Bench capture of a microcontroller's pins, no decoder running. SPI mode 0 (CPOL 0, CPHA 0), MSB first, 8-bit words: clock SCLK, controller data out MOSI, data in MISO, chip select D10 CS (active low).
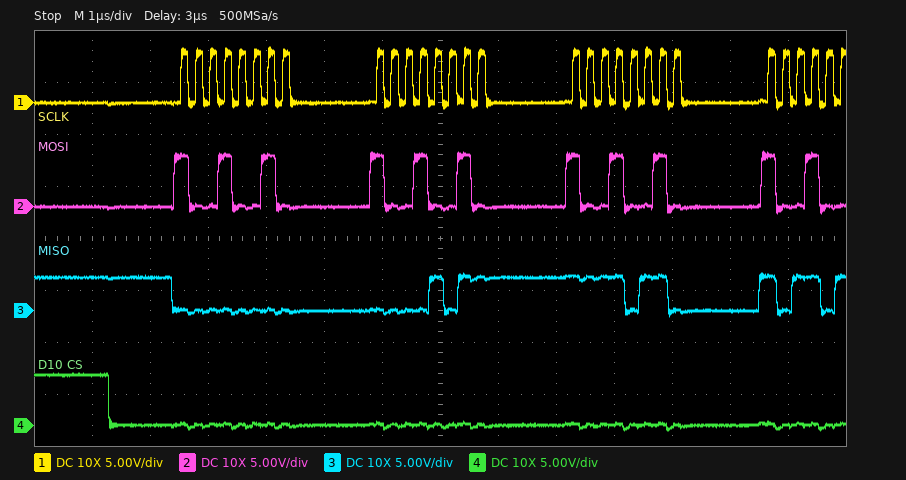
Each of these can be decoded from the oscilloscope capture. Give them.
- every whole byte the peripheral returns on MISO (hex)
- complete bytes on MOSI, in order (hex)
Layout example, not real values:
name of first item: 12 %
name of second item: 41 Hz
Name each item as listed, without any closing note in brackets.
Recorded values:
every whole byte the peripheral returns on MISO: 00 0B F6
complete bytes on MOSI, in order: 92 92 92
